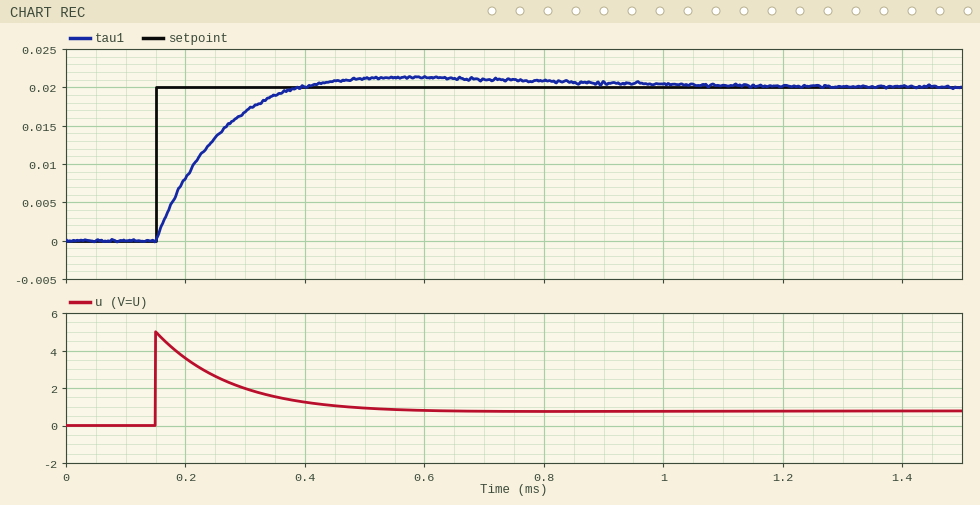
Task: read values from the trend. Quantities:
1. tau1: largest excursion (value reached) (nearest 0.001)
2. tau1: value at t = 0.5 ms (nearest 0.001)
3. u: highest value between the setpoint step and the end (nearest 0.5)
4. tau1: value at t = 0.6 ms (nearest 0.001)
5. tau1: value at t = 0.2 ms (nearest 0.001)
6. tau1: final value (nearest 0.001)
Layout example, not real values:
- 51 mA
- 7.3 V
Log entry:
- 0.021
- 0.021
- 5.0
- 0.021
- 0.008
- 0.020
